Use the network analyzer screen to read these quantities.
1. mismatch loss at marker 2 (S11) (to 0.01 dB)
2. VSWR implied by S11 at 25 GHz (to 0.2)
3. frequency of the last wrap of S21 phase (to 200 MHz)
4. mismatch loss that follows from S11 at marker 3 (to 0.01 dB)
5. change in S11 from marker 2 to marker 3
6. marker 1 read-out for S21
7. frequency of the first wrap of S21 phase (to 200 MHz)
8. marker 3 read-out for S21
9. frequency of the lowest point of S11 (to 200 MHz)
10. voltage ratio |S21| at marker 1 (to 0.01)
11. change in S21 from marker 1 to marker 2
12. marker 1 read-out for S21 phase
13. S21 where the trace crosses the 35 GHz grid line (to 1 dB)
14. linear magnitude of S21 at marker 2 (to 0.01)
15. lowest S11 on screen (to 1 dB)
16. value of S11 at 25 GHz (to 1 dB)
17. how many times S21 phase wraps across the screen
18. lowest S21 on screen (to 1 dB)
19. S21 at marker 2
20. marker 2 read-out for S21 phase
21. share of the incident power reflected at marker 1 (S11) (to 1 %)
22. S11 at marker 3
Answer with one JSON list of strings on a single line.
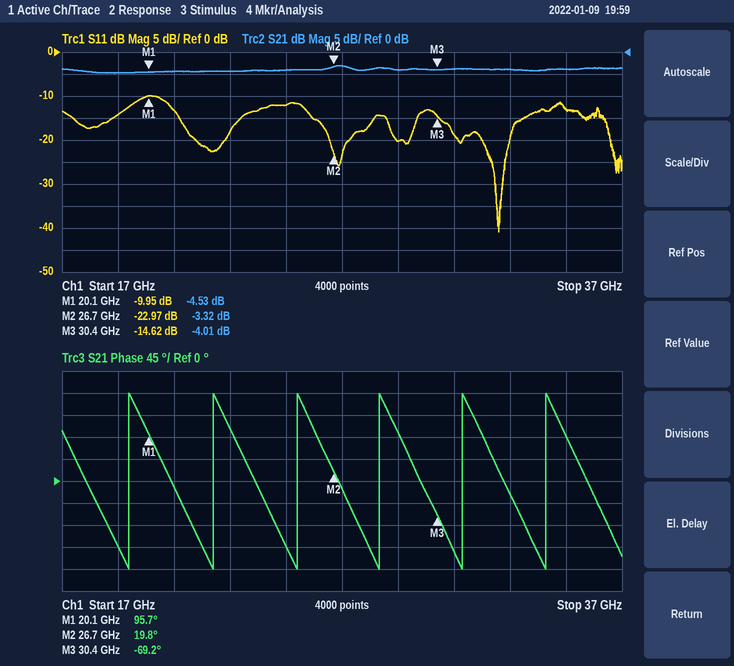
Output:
["0.02 dB", "1.6", "34.2 GHz", "0.15 dB", "8.35 dB", "-4.53 dB", "19.4 GHz", "-4.01 dB", "32.6 GHz", "0.59", "1.21 dB", "95.7°", "-4 dB", "0.68", "-41 dB", "-12 dB", "6", "-5 dB", "-3.32 dB", "19.8°", "10 %", "-14.62 dB"]
